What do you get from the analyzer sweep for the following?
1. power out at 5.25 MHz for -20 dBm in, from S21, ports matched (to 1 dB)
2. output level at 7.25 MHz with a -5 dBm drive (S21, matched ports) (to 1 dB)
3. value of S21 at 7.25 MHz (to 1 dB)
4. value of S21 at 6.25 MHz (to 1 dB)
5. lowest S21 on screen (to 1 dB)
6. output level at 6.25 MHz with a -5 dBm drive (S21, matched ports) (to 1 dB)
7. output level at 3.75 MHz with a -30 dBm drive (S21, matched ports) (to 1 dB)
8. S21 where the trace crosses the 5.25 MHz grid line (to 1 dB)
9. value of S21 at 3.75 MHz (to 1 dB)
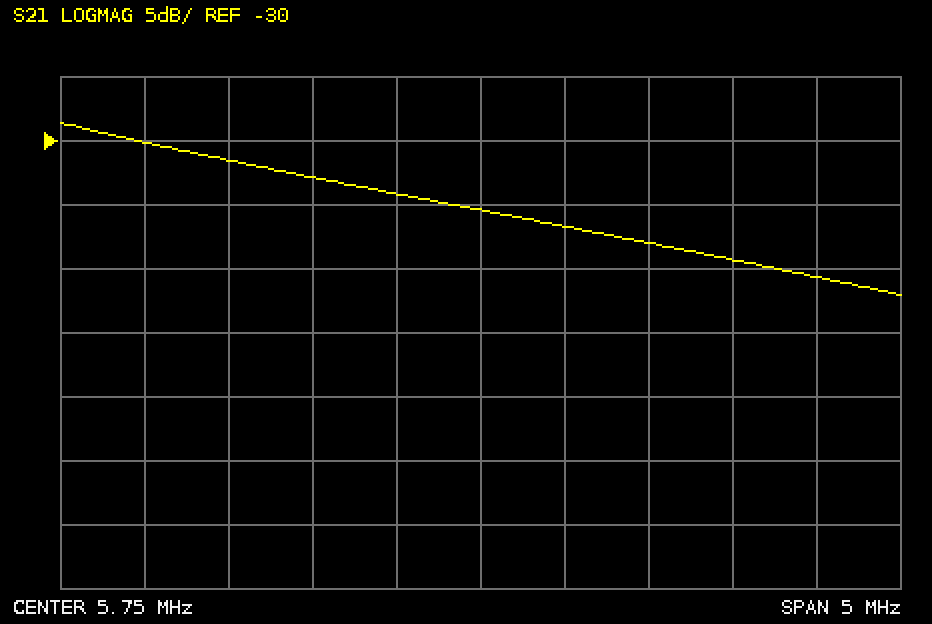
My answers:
-54 dBm
-44 dBm
-39 dB
-37 dB
-42 dB
-42 dBm
-60 dBm
-34 dB
-30 dB
